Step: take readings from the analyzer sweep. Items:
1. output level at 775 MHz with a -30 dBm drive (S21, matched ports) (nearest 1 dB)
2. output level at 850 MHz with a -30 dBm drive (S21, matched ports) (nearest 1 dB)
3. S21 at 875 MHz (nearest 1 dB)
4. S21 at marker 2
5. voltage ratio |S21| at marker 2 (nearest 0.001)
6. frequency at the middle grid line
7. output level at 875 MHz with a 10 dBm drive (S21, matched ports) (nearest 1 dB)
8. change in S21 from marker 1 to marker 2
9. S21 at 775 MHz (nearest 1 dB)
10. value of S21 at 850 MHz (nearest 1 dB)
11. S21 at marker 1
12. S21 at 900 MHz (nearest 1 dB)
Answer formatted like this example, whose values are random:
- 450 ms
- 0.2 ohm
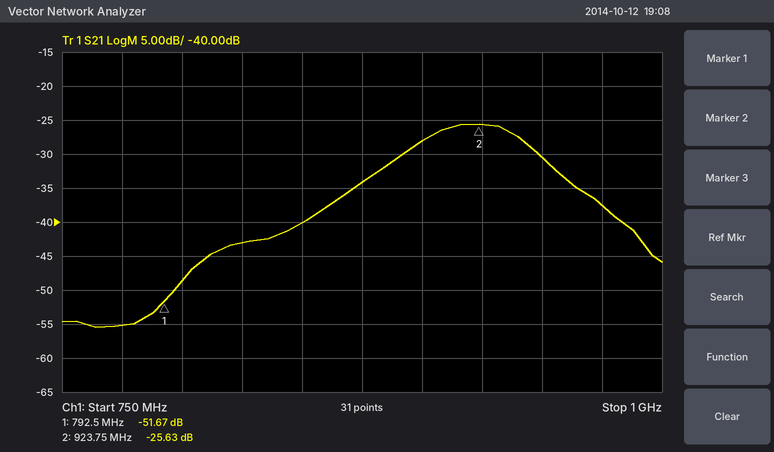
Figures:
- -85 dBm
- -70 dBm
- -34 dB
- -25.63 dB
- 0.052
- 875 MHz
- -24 dBm
- 26.04 dB
- -55 dB
- -40 dB
- -51.67 dB
- -28 dB
